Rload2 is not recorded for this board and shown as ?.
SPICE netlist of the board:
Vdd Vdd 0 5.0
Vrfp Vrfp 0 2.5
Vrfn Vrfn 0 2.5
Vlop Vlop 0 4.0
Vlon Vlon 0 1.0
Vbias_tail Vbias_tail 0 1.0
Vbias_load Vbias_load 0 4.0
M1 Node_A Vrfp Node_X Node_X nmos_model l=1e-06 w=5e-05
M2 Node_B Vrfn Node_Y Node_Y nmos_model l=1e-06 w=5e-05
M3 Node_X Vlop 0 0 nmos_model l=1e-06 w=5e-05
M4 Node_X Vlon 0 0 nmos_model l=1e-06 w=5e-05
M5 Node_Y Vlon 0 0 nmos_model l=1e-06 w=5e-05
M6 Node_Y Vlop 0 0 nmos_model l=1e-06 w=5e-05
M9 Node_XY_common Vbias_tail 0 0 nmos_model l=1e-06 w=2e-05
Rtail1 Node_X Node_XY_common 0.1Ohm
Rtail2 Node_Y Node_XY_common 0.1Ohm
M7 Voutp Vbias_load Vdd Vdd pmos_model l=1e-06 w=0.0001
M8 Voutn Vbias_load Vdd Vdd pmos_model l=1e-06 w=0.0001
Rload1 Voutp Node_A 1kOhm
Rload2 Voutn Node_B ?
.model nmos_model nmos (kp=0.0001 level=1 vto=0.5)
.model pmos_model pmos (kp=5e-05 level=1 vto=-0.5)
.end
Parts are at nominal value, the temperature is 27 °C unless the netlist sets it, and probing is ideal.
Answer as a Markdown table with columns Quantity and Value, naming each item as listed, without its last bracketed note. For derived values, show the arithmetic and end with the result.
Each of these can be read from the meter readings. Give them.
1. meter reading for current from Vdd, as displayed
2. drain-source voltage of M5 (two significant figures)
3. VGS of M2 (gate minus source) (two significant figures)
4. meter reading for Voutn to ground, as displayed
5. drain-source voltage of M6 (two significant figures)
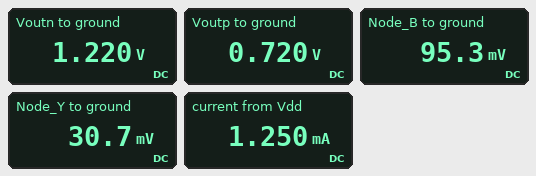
| Quantity | Value |
|---|---|
| meter reading for current from Vdd, as displayed | 1.250 mA |
| drain-source voltage of M5 | 30.7 mV = 31 mV |
| VGS of M2 (gate minus source) | 2.5 V - 30.7 mV = 2.5 V |
| meter reading for Voutn to ground, as displayed | 1.220 V |
| drain-source voltage of M6 | 30.7 mV = 31 mV |
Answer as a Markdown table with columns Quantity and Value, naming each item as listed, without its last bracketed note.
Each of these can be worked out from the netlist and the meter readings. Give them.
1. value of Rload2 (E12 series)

| Quantity | Value |
|---|---|
| value of Rload2 | 1.8 kΩ |
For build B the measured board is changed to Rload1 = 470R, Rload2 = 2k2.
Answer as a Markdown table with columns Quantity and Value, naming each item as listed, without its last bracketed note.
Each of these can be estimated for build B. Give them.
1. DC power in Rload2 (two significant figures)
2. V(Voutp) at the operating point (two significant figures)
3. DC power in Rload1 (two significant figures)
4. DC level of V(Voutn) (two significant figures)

| Quantity | Value |
|---|---|
| DC power in Rload2 | 860 µW |
| V(Voutp) at the operating point | 390 mV |
| DC power in Rload1 | 180 µW |
| DC level of V(Voutn) | 1.5 V |
